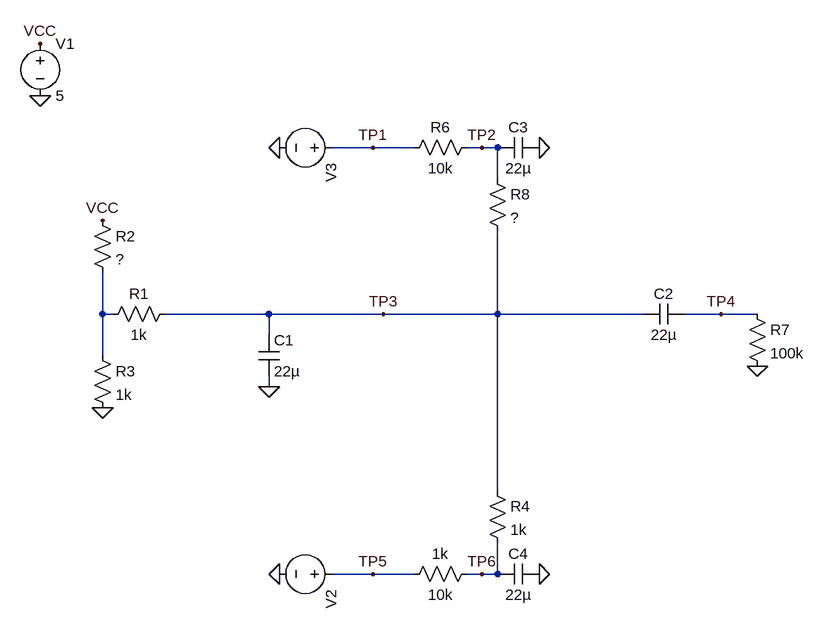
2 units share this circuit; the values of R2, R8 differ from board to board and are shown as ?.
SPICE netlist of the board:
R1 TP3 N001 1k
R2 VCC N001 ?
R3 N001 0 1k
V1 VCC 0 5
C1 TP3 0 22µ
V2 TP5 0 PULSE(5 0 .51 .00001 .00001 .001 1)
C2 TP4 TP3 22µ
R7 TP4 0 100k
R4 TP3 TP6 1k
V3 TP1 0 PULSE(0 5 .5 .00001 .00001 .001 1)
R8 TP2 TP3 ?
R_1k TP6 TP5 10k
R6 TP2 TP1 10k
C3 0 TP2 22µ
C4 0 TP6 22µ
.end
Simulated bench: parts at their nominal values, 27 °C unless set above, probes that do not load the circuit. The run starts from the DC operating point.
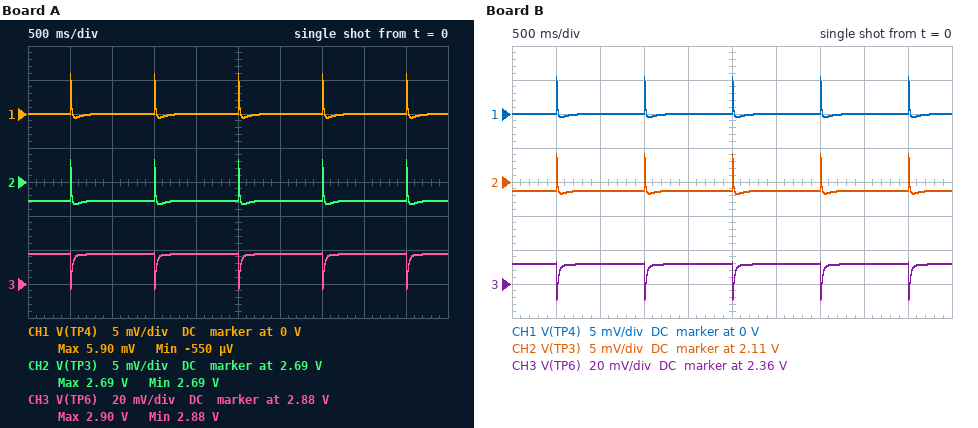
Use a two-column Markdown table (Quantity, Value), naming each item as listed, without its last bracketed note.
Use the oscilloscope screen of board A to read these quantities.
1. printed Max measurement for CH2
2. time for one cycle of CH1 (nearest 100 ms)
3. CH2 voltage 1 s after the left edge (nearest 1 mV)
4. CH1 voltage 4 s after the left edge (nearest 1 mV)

| Quantity | Value |
|---|---|
| printed Max measurement for CH2 | 2.69 V |
| time for one cycle of CH1 | 1.0 s |
| CH2 voltage 1 s after the left edge | 2.687 V |
| CH1 voltage 4 s after the left edge | 0 V |
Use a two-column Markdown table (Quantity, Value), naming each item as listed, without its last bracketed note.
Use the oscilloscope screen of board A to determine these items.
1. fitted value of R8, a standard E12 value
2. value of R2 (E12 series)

| Quantity | Value |
|---|---|
| fitted value of R8, a standard E12 value | 680 Ω |
| value of R2 | 820 Ω |
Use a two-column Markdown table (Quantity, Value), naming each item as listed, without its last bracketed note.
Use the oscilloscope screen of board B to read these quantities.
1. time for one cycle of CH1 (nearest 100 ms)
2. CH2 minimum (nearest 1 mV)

| Quantity | Value |
|---|---|
| time for one cycle of CH1 | 1.0 s |
| CH2 minimum | 2.108 V |
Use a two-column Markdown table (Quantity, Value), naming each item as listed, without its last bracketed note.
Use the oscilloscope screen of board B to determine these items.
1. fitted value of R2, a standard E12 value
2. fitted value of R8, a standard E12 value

| Quantity | Value |
|---|---|
| fitted value of R2, a standard E12 value | 1.5 kΩ |
| fitted value of R8, a standard E12 value | 820 Ω |
